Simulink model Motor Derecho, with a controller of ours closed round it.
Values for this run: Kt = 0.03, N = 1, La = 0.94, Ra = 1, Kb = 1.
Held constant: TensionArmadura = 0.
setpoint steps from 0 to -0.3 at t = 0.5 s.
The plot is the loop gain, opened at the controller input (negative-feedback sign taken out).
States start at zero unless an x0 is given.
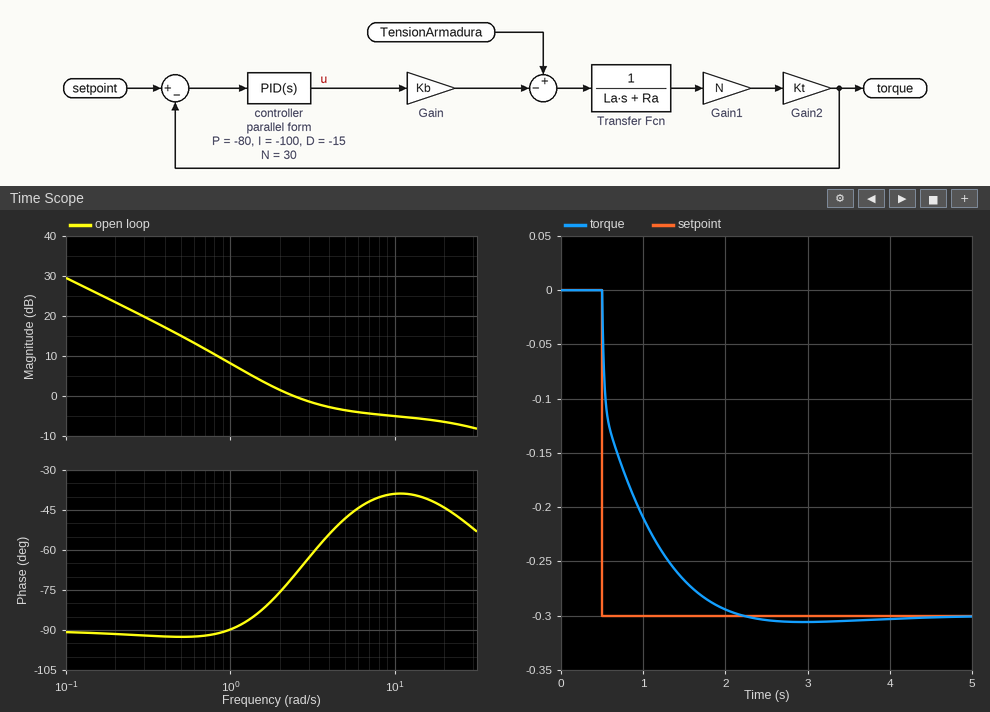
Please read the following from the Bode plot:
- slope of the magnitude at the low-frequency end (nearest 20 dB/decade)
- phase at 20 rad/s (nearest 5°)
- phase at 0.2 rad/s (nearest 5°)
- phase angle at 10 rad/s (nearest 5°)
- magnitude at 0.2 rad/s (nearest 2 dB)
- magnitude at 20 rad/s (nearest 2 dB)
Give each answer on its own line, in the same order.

-20 dB/decade
-45°
-90°
-40°
24 dB
-6 dB
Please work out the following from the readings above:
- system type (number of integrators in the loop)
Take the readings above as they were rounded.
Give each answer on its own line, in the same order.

1
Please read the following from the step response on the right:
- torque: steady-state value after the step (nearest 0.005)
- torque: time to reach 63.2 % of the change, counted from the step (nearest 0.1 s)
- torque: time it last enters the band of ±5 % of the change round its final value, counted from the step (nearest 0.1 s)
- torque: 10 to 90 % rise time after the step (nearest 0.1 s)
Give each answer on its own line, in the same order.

-0.300
0.4 s
1.3 s
1.0 s
